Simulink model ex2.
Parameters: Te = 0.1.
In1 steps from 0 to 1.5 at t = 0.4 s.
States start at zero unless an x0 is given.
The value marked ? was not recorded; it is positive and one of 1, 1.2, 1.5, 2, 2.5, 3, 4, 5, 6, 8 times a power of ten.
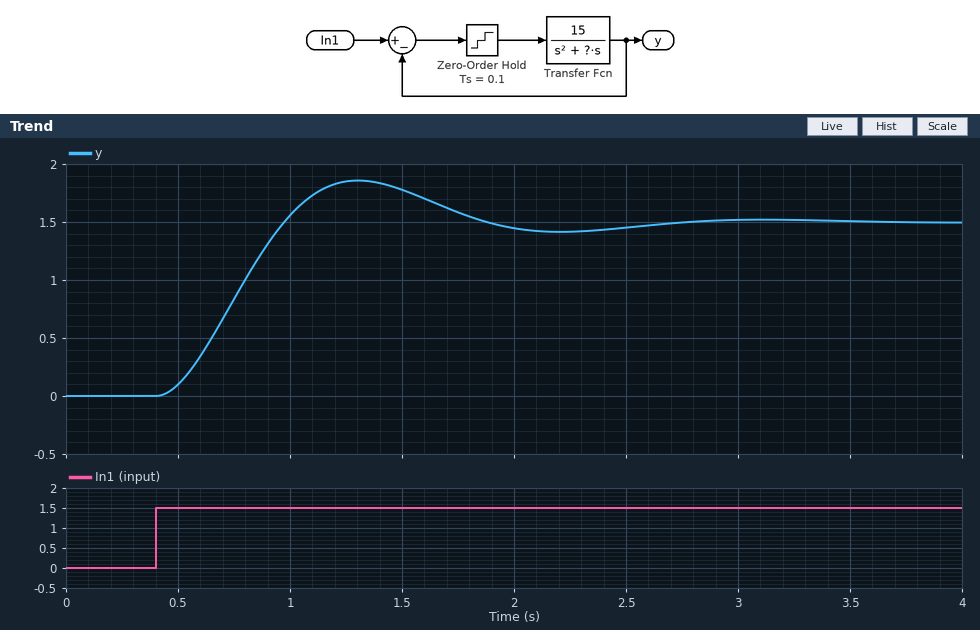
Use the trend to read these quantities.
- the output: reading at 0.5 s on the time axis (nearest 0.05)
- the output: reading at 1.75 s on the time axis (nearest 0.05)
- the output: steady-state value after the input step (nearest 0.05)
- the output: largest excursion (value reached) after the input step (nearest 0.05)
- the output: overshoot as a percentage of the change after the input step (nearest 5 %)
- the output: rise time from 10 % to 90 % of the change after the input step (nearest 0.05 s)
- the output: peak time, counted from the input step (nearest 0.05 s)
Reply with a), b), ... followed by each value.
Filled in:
a) 0.10
b) 1.60
c) 1.50
d) 1.85
e) 25 %
f) 0.40 s
g) 0.90 s
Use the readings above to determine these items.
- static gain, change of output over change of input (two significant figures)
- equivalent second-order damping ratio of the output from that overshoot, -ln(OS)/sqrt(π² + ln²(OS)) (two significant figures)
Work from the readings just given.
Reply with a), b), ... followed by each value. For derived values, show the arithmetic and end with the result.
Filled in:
a) (1.5 - 0) / (1.5 - 0) = 1.0
b) ln(0.25) = -1.386; 1.386 / sqrt(9.870 + 1.922) = 0.40
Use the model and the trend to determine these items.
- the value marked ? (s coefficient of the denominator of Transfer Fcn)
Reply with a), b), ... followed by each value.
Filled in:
a) 4
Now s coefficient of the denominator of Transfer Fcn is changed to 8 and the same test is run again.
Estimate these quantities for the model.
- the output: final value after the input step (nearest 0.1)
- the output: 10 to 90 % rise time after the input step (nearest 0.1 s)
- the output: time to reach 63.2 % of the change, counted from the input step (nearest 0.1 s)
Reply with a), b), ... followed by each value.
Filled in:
a) 1.5
b) 0.8 s
c) 0.5 s
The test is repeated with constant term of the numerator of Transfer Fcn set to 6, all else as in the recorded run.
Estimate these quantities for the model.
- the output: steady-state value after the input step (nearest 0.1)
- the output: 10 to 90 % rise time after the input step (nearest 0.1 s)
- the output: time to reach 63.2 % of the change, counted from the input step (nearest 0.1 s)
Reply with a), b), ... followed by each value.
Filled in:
a) 1.5
b) 0.9 s
c) 0.7 s
